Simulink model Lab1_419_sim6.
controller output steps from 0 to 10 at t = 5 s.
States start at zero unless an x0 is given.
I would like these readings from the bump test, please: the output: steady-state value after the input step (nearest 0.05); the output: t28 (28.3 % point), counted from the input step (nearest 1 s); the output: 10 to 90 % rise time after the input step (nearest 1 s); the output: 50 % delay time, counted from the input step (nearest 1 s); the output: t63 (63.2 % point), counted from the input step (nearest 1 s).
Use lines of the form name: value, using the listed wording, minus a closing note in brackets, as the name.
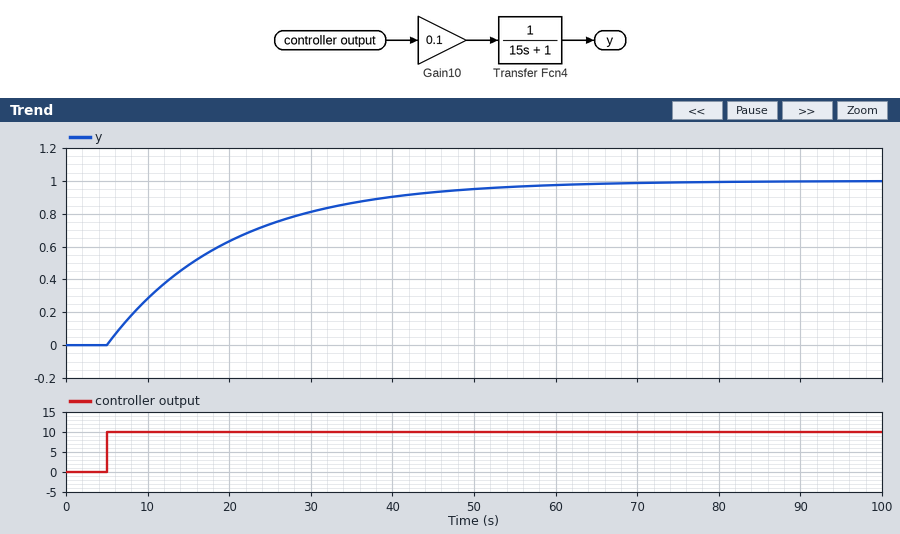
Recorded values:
the output: steady-state value after the input step: 1.00
the output: t28 (28.3 % point), counted from the input step: 5 s
the output: 10 to 90 % rise time after the input step: 33 s
the output: 50 % delay time, counted from the input step: 10 s
the output: t63 (63.2 % point), counted from the input step: 15 s
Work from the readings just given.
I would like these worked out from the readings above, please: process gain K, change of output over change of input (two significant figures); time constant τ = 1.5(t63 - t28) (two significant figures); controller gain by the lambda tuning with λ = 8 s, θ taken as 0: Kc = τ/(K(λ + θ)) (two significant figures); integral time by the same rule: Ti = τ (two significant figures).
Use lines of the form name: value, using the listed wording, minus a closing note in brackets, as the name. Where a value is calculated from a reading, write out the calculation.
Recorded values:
process gain K, change of output over change of input: (1 - 0) / 10 = 0.10
time constant τ = 1.5(t63 - t28): 1.5 × (15 - 5) = 15 s
controller gain by the lambda tuning with λ = 8 s, θ taken as 0: Kc = τ/(K(λ + θ)): 15 / (0.1 × (8 + 0)) = 19
integral time by the same rule: Ti = τ: 15 s
